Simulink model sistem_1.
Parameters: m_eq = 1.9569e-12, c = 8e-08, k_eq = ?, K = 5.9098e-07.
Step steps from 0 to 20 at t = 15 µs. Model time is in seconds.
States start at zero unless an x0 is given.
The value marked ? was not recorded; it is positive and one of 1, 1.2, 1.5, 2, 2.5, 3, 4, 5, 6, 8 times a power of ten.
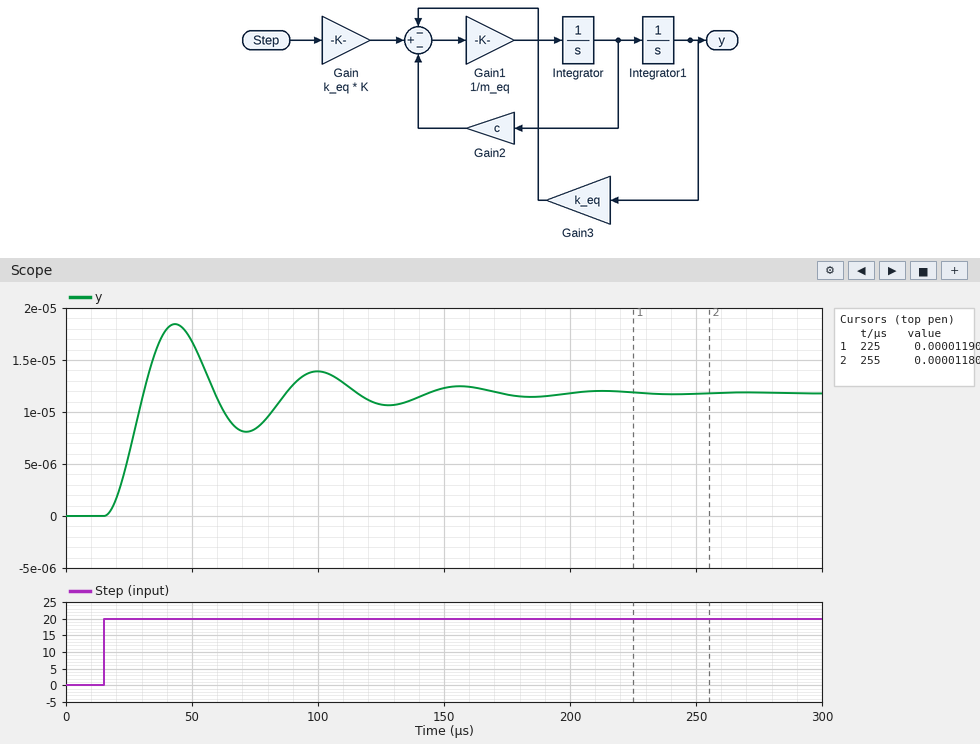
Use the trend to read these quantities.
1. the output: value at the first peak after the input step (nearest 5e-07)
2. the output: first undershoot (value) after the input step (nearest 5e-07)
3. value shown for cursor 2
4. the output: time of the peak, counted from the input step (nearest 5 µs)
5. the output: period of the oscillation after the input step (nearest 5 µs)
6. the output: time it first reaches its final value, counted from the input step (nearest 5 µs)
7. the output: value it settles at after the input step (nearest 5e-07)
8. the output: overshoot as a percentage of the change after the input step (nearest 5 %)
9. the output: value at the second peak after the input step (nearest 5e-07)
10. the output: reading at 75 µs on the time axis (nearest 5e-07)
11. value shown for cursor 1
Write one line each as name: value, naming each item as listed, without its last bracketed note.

the output: value at the first peak after the input step: 0.0000185
the output: first undershoot (value) after the input step: 0.0000080
value shown for cursor 2: 0.00001180
the output: time of the peak, counted from the input step: 30 µs
the output: period of the oscillation after the input step: 55 µs
the output: time it first reaches its final value, counted from the input step: 15 µs
the output: value it settles at after the input step: 0.0000120
the output: overshoot as a percentage of the change after the input step: 55 %
the output: value at the second peak after the input step: 0.0000140
the output: reading at 75 µs on the time axis: 0.0000085
value shown for cursor 1: 0.00001190
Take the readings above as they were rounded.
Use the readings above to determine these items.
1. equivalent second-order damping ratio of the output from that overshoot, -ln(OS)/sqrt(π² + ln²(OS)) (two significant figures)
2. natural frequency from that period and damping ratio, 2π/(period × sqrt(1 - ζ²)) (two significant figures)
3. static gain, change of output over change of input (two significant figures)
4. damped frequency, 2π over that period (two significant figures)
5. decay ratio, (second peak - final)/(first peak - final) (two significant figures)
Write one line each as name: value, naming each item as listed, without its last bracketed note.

equivalent second-order damping ratio of the output from that overshoot, -ln(OS)/sqrt(π² + ln²(OS)): 0.19
natural frequency from that period and damping ratio, 2π/(period × sqrt(1 - ζ²)): 0.12 rad/µs
static gain, change of output over change of input: 0.00000060
damped frequency, 2π over that period: 0.11 rad/µs
decay ratio, (second peak - final)/(first peak - final): 0.31
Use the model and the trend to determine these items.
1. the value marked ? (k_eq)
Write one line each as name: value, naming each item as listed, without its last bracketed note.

the value marked ?: 0.025
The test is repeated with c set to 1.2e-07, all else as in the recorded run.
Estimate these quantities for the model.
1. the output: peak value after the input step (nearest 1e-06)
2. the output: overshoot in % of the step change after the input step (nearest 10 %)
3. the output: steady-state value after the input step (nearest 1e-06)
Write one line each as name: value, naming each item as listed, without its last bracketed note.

the output: peak value after the input step: 0.000017
the output: overshoot in % of the step change after the input step: 40 %
the output: steady-state value after the input step: 0.000012
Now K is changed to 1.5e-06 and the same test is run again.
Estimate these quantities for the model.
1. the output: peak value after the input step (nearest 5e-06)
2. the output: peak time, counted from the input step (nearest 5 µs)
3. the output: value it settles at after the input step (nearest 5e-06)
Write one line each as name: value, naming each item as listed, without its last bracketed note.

the output: peak value after the input step: 0.000045
the output: peak time, counted from the input step: 30 µs
the output: value it settles at after the input step: 0.000030
